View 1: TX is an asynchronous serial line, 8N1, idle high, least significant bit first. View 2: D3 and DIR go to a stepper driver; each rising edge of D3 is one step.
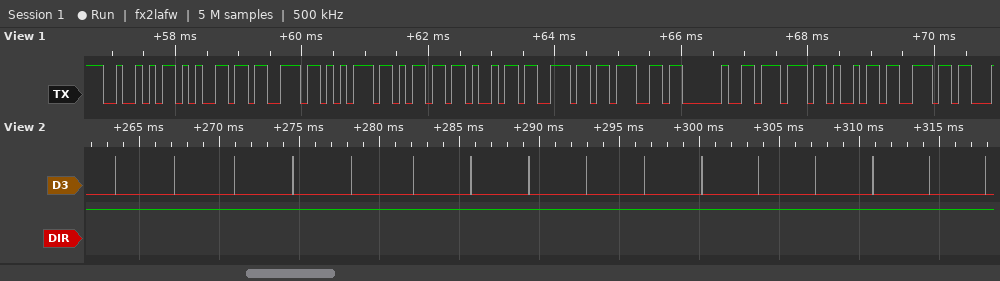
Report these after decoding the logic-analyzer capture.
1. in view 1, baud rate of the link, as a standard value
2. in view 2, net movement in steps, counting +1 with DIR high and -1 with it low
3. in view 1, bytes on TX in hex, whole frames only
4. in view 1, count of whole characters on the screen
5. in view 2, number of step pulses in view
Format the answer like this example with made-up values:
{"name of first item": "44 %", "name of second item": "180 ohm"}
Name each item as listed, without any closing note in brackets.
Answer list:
{"in view 1, baud rate of the link, as a standard value": "9600 baud", "in view 2, net movement in steps, counting +1 with DIR high and -1 with it low": "+16", "in view 1, bytes on TX in hex, whole frames only": "52 65 73 75 6D 69 6E 67 20 77 69 6E", "in view 1, count of whole characters on the screen": "12", "in view 2, number of step pulses in view": "16"}
